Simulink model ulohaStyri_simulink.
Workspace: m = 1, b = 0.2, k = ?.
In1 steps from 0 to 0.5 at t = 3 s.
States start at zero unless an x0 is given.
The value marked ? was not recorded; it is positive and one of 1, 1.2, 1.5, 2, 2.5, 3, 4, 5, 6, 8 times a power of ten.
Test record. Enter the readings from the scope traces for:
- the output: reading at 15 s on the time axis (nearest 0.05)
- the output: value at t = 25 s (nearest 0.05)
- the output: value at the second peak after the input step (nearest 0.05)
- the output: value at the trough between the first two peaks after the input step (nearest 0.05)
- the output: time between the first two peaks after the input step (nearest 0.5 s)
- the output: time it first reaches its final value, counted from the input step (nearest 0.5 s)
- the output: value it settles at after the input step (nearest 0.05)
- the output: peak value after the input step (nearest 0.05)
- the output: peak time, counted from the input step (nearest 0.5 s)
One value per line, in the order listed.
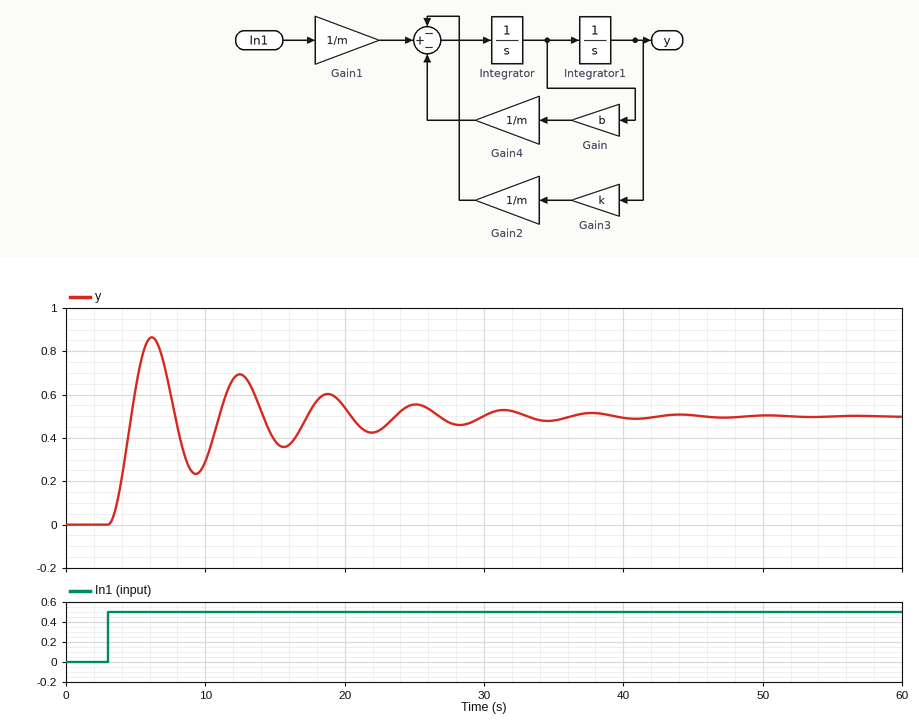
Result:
0.40
0.55
0.70
0.25
6.5 s
1.5 s
0.50
0.85
3.0 s
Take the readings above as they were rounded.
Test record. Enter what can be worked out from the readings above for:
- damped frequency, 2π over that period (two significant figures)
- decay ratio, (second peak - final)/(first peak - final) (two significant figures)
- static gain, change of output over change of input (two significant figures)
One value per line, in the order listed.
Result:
0.97 rad/s
0.57
1.0
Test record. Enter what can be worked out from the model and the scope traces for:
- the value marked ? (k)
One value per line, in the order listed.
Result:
1
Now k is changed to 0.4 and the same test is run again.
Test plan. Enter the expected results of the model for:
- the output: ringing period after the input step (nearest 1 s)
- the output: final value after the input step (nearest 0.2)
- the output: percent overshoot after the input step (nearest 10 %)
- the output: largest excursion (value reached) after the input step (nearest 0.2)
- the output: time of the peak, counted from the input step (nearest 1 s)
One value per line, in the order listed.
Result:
10 s
1.2
60 %
2.0
5 s
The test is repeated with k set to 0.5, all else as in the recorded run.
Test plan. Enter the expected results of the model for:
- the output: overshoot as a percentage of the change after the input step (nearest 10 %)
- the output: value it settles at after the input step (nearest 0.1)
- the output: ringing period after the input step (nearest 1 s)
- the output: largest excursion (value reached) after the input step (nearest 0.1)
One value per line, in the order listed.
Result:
60 %
1.0
9 s
1.6
